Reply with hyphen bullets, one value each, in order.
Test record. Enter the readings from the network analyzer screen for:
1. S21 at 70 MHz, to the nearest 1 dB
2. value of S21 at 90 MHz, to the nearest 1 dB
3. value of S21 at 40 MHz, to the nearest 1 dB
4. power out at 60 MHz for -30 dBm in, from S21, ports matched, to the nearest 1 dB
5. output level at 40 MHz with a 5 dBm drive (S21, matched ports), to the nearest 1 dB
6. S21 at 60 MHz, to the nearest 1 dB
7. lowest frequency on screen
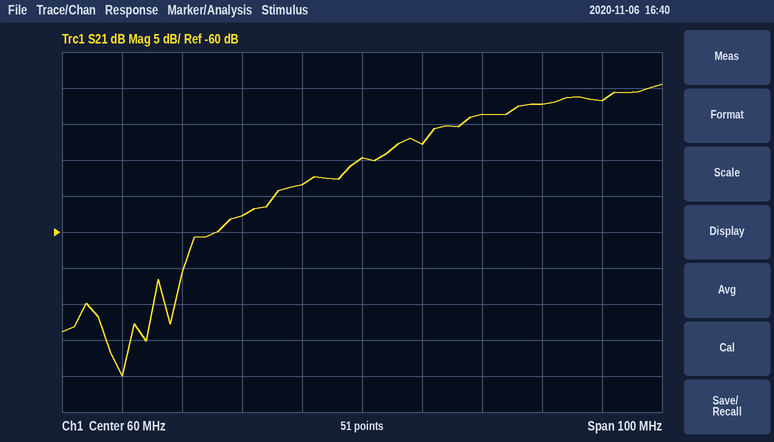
- -48 dB
- -42 dB
- -58 dB
- -80 dBm
- -53 dBm
- -50 dB
- 10 MHz
